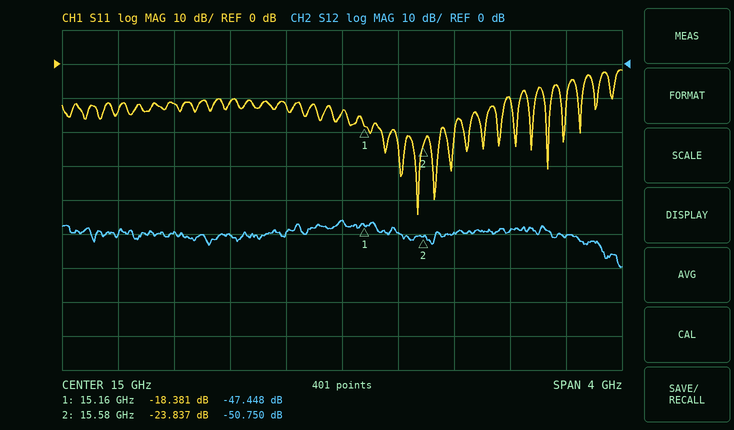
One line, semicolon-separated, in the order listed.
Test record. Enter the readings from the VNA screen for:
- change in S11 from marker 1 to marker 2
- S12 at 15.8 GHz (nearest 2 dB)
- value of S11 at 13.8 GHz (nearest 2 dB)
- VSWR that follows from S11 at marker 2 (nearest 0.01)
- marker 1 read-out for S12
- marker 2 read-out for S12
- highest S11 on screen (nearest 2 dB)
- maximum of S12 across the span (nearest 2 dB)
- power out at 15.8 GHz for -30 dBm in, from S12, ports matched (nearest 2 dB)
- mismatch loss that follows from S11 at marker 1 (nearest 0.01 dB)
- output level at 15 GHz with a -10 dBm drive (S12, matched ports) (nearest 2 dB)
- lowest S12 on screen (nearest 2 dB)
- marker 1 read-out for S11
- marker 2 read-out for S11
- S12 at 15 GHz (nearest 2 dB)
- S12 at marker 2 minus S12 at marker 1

-5.456 dB; -50 dB; -12 dB; 1.14; -47.448 dB; -50.750 dB; -2 dB; -46 dB; -80 dBm; 0.06 dB; -56 dBm; -60 dB; -18.381 dB; -23.837 dB; -46 dB; -3.302 dB
